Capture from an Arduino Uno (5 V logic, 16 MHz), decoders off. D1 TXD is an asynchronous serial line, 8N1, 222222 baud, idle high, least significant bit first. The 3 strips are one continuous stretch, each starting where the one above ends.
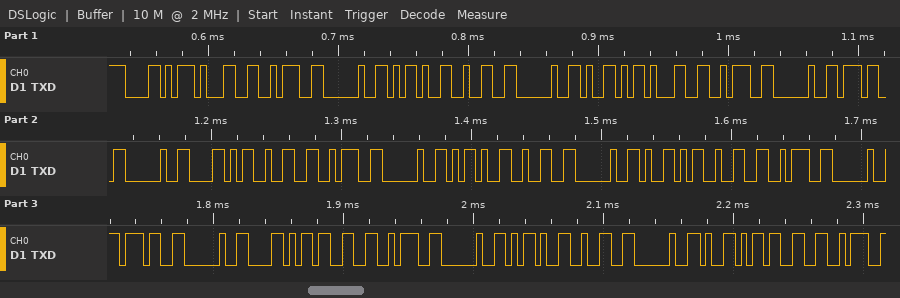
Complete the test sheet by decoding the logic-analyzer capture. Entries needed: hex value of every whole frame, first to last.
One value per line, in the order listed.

58 31 3A 20 2D 32 20 59 31 3A 20 37 20 58 32 3A 20 2D 32 20 59 32 3A 20 37 20 58 33 3A 20 2D 32 20 59 33 3A
